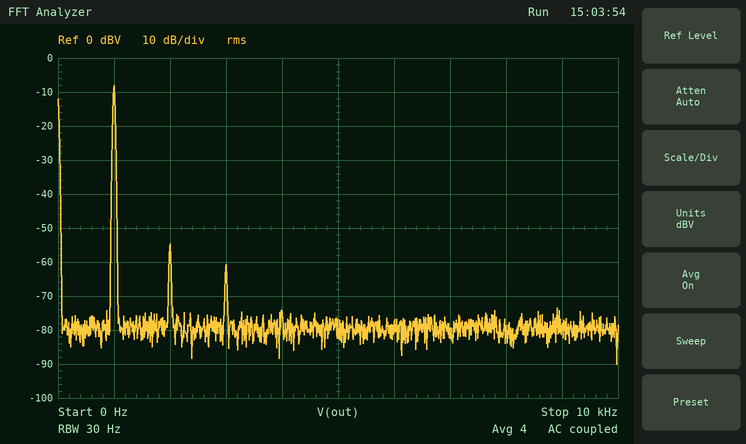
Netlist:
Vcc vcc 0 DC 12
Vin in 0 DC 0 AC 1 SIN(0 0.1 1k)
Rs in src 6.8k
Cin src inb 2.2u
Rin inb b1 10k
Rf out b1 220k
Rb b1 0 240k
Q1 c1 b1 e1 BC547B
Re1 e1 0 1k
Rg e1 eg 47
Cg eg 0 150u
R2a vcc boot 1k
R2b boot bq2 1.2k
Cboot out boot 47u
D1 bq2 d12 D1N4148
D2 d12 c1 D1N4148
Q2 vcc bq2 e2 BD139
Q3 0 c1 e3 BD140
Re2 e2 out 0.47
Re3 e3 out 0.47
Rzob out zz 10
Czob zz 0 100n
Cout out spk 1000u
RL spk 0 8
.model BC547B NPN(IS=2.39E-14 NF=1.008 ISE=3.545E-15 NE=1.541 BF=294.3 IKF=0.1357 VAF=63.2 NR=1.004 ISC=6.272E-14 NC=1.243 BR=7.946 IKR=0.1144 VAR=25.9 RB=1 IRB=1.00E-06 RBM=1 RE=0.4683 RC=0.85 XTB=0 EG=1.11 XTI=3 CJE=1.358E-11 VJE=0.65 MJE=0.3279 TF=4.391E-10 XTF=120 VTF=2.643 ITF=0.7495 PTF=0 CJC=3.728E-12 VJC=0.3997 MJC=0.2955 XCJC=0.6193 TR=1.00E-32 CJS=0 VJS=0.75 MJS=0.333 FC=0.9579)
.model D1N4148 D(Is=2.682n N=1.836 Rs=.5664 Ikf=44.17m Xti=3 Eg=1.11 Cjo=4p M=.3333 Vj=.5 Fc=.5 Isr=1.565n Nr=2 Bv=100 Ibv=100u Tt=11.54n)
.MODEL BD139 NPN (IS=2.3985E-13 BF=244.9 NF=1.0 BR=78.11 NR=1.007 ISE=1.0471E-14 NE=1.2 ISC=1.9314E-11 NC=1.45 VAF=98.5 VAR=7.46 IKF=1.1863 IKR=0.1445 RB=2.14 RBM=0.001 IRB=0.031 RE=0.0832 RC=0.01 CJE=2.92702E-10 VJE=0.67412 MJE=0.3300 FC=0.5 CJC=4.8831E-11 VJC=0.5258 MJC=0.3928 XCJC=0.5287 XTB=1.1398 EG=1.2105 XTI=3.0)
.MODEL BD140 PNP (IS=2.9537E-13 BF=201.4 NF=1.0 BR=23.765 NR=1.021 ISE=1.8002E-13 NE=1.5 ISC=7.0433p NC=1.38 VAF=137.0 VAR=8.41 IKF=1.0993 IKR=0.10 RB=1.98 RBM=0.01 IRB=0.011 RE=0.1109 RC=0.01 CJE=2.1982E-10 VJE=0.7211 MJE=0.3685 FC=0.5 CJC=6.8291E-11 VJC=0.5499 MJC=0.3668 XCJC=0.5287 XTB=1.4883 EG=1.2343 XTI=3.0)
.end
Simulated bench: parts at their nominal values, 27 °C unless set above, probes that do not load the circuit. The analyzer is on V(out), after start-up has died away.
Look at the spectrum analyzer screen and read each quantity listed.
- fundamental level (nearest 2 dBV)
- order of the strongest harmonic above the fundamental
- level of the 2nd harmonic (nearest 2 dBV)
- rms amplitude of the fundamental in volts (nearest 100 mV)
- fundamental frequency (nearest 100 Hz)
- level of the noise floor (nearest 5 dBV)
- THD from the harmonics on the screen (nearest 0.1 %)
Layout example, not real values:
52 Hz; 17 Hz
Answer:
-8 dBV; 2; -54 dBV; 400 mV; 1.0 kHz; -80 dBV; 0.5 %
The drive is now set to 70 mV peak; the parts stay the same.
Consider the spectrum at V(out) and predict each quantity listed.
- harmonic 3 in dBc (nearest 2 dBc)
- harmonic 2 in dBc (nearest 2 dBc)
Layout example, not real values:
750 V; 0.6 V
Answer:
-58 dBc; -48 dBc
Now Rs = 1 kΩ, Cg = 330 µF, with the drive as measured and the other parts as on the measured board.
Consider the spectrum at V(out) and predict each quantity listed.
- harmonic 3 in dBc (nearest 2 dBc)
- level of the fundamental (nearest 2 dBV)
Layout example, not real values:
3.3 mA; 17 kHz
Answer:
-48 dBc; -6 dBV
